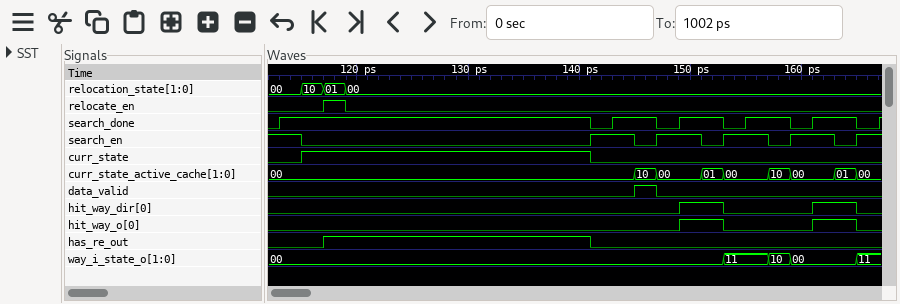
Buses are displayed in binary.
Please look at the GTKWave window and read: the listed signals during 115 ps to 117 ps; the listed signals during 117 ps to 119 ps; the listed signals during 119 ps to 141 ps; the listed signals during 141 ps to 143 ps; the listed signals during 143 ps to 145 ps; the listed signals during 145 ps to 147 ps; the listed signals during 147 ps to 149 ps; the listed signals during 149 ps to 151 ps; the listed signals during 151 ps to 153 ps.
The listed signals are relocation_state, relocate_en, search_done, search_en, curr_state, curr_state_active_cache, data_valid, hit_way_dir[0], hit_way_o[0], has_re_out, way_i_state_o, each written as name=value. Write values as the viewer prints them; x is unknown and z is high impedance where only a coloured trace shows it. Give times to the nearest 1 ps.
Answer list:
relocation_state=10, relocate_en=0, search_done=1, search_en=0, curr_state=1, curr_state_active_cache=00, data_valid=0, hit_way_dir[0]=0, hit_way_o[0]=0, has_re_out=0, way_i_state_o=00
relocation_state=01, relocate_en=1, search_done=1, search_en=0, curr_state=1, curr_state_active_cache=00, data_valid=0, hit_way_dir[0]=0, hit_way_o[0]=0, has_re_out=1, way_i_state_o=00
relocation_state=00, relocate_en=0, search_done=1, search_en=0, curr_state=1, curr_state_active_cache=00, data_valid=0, hit_way_dir[0]=0, hit_way_o[0]=0, has_re_out=1, way_i_state_o=00
relocation_state=00, relocate_en=0, search_done=0, search_en=1, curr_state=0, curr_state_active_cache=00, data_valid=0, hit_way_dir[0]=0, hit_way_o[0]=0, has_re_out=0, way_i_state_o=00
relocation_state=00, relocate_en=0, search_done=1, search_en=1, curr_state=0, curr_state_active_cache=00, data_valid=0, hit_way_dir[0]=0, hit_way_o[0]=0, has_re_out=0, way_i_state_o=00
relocation_state=00, relocate_en=0, search_done=1, search_en=0, curr_state=0, curr_state_active_cache=10, data_valid=1, hit_way_dir[0]=0, hit_way_o[0]=0, has_re_out=0, way_i_state_o=00
relocation_state=00, relocate_en=0, search_done=0, search_en=1, curr_state=0, curr_state_active_cache=00, data_valid=0, hit_way_dir[0]=0, hit_way_o[0]=0, has_re_out=0, way_i_state_o=00
relocation_state=00, relocate_en=0, search_done=1, search_en=1, curr_state=0, curr_state_active_cache=00, data_valid=0, hit_way_dir[0]=1, hit_way_o[0]=1, has_re_out=0, way_i_state_o=00
relocation_state=00, relocate_en=0, search_done=1, search_en=0, curr_state=0, curr_state_active_cache=01, data_valid=0, hit_way_dir[0]=1, hit_way_o[0]=1, has_re_out=0, way_i_state_o=00
